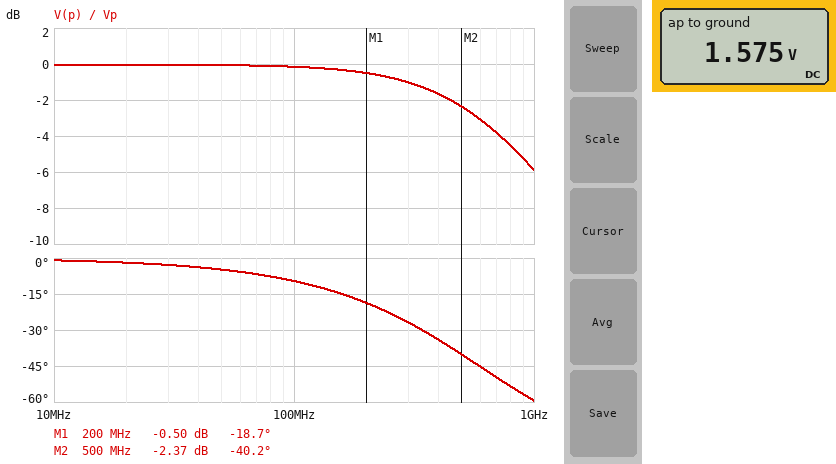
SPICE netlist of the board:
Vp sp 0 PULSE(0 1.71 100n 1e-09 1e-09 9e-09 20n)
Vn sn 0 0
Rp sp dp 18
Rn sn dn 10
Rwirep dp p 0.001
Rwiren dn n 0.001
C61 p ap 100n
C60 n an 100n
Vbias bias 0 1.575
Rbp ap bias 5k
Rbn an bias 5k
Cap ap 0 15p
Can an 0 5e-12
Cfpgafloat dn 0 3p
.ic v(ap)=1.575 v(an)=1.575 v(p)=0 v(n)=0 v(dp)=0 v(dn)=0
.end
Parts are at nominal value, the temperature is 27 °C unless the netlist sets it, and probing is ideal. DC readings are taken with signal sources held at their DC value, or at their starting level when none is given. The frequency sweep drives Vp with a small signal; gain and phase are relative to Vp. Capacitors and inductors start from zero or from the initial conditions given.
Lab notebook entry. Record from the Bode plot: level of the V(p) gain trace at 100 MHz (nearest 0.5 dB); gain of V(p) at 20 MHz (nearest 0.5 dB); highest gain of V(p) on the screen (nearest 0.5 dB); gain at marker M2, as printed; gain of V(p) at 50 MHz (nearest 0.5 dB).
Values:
0 dB
0 dB
0 dB
-2.37 dB
0 dB
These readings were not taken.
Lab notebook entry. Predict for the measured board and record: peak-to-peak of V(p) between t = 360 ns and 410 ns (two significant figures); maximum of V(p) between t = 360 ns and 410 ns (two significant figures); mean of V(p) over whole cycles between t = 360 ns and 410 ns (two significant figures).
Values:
1.7 V
1.7 V
850 mV
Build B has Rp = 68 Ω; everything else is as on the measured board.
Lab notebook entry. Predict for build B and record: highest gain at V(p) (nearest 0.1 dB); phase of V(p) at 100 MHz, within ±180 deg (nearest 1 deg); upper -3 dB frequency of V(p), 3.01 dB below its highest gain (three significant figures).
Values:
-0.1 dB
-32 deg
158 MHz
